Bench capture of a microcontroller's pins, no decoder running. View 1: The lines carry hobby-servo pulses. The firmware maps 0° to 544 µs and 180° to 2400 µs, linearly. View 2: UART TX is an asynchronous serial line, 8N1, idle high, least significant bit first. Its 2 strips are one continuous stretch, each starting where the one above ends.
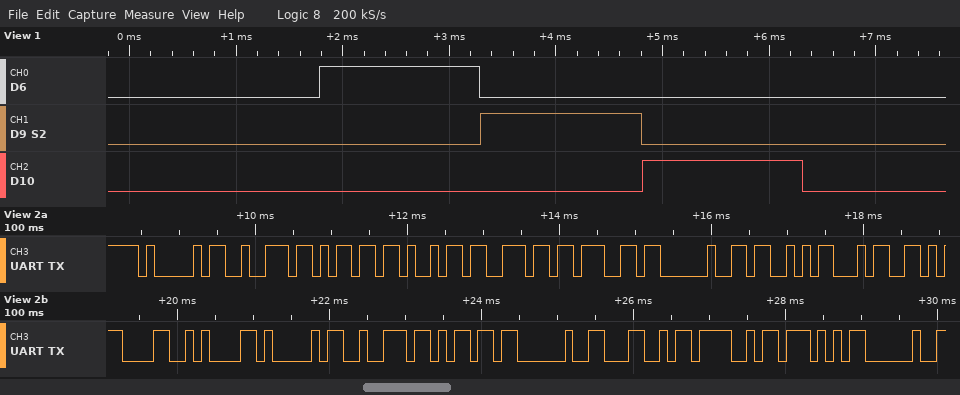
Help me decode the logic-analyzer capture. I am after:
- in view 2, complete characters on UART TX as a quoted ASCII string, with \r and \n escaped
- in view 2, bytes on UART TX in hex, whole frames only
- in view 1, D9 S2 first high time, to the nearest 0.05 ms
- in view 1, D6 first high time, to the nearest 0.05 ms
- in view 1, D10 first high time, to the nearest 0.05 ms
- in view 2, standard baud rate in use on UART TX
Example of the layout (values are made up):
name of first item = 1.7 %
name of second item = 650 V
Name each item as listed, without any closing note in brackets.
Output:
in view 2, complete characters on UART TX as a quoted ASCII string, with \r and \n escaped = "Arming S4\r\nArm LOW "
in view 2, bytes on UART TX in hex, whole frames only = 41 72 6D 69 6E 67 20 53 34 0D 0A 41 72 6D 20 4C 4F 57 20
in view 1, D9 S2 first high time, to the nearest 0.05 ms = 1.50 ms
in view 1, D6 first high time, to the nearest 0.05 ms = 1.50 ms
in view 1, D10 first high time, to the nearest 0.05 ms = 1.50 ms
in view 2, standard baud rate in use on UART TX = 9600 baud
